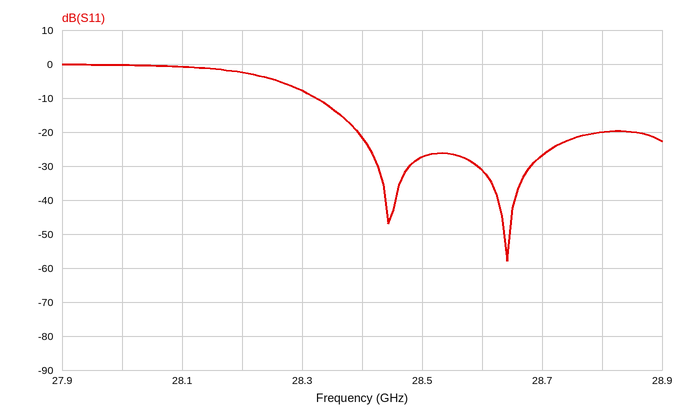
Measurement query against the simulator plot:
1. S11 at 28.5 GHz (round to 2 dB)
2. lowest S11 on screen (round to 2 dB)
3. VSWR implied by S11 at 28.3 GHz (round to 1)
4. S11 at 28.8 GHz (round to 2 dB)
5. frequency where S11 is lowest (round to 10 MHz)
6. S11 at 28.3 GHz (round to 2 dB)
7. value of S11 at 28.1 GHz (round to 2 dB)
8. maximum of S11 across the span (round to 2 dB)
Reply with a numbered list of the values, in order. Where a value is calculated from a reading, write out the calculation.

1. -28 dB
2. -58 dB
3. |Γ| = 10^(-8/20) = 0.3981; VSWR = (1 + 0.3981)/(1 − 0.3981) ≈ 2
4. -20 dB
5. 28.64 GHz
6. -8 dB
7. 0 dB
8. 0 dB
